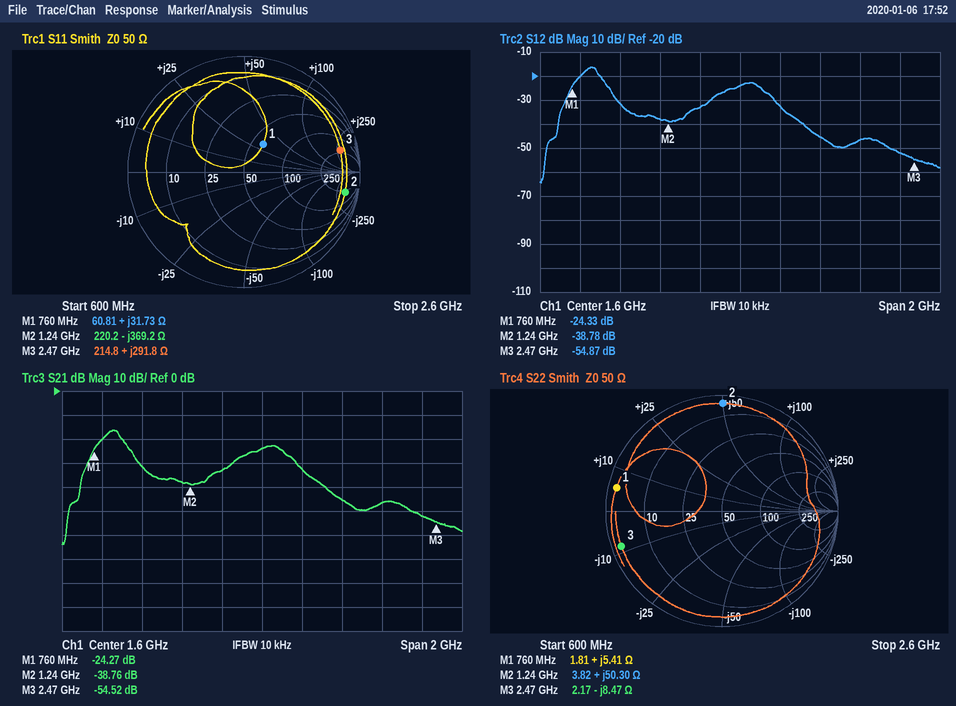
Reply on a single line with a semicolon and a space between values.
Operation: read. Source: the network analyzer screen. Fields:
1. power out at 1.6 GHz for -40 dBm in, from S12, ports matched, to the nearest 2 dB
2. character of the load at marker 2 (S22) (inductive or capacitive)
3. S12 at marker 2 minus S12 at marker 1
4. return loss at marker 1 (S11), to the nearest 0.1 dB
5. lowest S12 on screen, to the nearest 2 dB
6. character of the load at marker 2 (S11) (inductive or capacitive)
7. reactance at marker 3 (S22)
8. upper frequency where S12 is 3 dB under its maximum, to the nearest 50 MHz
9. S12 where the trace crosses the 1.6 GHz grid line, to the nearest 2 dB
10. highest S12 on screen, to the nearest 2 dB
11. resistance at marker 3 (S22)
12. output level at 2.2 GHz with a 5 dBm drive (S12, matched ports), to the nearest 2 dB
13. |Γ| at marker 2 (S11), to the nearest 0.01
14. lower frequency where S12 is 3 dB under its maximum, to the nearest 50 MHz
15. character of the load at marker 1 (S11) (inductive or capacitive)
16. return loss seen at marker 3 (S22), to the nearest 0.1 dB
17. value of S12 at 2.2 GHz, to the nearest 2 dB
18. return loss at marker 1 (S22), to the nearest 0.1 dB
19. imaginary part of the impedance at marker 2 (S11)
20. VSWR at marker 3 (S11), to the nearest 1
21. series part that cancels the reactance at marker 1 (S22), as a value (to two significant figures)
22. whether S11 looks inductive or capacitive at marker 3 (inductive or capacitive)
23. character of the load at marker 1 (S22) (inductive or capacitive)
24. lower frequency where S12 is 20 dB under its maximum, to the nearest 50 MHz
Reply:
-64 dBm; inductive; -14.45 dB; 10.7 dB; -64 dB; capacitive; -8.47 Ω; 900 MHz; -24 dB; -16 dB; 2.17 Ω; -42 dBm; 0.89; 800 MHz; inductive; 0.7 dB; -46 dB; 0.6 dB; -369.2 Ω; 12; 39 pF; inductive; inductive; 700 MHz
